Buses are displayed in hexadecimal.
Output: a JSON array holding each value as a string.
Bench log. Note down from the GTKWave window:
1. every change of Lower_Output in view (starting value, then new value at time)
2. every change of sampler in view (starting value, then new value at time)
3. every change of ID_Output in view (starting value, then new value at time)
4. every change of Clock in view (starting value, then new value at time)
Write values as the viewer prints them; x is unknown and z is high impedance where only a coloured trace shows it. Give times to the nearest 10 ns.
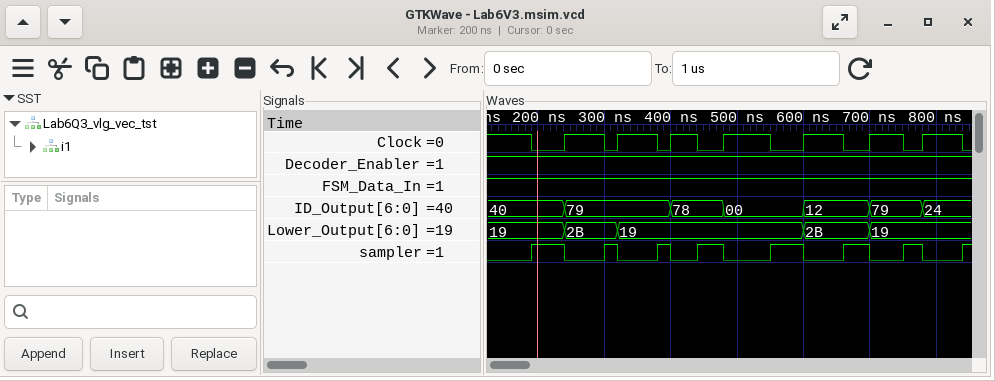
["19, 2B at 240 ns, 19 at 320 ns, 2B at 600 ns, 19 at 700 ns", "0, 1 at 190 ns, 0 at 240 ns, 1 at 300 ns, 0 at 320 ns, 1 at 380 ns, 0 at 400 ns, 1 at 440 ns, 0 at 480 ns, 1 at 550 ns, 0 at 600 ns, 1 at 660 ns, 0 at 700 ns, 1 at 750 ns, 0 at 780 ns, 1 at 840 ns", "40, 79 at 240 ns, 78 at 400 ns, 00 at 480 ns, 12 at 600 ns, 79 at 700 ns, 24 at 780 ns", "1, 0 at 190 ns, 1 at 240 ns, 0 at 300 ns, 1 at 320 ns, 0 at 380 ns, 1 at 400 ns, 0 at 440 ns, 1 at 480 ns, 0 at 550 ns, 1 at 600 ns, 0 at 660 ns, 1 at 700 ns, 0 at 750 ns, 1 at 780 ns, 0 at 840 ns"]
